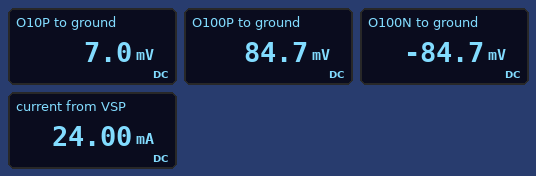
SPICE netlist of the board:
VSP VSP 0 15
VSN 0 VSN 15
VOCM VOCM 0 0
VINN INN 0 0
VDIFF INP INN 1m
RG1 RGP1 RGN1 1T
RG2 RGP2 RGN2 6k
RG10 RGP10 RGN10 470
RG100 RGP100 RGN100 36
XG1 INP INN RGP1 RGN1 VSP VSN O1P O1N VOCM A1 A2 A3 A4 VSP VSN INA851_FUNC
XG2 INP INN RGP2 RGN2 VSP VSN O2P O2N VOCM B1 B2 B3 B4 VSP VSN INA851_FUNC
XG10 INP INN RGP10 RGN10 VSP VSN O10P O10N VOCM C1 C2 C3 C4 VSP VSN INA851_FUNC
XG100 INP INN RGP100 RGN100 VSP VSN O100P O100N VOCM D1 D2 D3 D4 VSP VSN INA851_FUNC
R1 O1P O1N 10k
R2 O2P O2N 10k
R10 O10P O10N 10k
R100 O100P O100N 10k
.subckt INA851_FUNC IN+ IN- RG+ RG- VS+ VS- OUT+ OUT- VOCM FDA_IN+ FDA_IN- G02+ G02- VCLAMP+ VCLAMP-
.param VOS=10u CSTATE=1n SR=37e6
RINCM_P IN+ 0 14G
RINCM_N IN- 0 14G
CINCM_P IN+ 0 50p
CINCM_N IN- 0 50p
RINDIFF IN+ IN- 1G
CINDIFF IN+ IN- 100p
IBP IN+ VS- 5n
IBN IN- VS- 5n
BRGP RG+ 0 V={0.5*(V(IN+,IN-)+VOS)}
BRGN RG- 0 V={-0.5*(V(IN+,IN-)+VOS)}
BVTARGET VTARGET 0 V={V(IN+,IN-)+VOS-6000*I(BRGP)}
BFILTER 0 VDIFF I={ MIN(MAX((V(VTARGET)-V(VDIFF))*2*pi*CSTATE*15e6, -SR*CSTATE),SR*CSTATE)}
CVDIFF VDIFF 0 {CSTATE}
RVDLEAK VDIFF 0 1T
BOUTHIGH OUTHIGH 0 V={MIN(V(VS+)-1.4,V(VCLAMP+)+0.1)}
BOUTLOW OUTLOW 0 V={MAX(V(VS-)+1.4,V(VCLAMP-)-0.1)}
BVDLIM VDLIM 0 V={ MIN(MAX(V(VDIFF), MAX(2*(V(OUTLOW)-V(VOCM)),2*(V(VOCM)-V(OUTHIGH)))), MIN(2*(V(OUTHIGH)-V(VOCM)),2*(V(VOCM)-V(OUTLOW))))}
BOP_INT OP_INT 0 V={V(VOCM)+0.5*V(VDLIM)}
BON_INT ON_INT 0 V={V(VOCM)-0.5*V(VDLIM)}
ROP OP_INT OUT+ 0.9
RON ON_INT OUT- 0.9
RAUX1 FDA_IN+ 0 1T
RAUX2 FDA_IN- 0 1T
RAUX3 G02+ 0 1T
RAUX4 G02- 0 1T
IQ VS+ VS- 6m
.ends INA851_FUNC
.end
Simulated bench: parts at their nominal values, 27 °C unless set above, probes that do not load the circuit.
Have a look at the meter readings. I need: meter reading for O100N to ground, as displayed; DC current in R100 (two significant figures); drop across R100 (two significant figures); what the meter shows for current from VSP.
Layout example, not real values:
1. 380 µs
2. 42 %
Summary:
1. -84.7 mV
2. 17 µA
3. 170 mV
4. 24.00 mA
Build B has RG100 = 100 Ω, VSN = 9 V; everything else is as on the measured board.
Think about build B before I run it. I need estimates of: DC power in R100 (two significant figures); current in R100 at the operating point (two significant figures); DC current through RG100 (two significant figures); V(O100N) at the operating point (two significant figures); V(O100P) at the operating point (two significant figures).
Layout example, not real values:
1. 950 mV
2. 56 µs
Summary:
1. 380 nW
2. 6.2 µA
3. 10 µA
4. -31 mV
5. 31 mV
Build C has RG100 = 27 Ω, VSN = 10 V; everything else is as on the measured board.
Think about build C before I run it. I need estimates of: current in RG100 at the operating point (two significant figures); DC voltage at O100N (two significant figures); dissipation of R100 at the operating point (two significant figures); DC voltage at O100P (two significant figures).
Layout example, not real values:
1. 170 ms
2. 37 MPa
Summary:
1. 37 µA
2. -110 mV
3. 5.1 µW
4. 110 mV
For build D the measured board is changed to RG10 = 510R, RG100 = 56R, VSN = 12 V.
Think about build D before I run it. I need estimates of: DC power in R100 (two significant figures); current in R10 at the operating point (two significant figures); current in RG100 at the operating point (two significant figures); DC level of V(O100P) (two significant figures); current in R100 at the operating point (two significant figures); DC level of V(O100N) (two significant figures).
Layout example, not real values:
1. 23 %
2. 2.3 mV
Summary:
1. 1.2 µW
2. 1.3 µA
3. 18 µA
4. 55 mV
5. 11 µA
6. -55 mV
